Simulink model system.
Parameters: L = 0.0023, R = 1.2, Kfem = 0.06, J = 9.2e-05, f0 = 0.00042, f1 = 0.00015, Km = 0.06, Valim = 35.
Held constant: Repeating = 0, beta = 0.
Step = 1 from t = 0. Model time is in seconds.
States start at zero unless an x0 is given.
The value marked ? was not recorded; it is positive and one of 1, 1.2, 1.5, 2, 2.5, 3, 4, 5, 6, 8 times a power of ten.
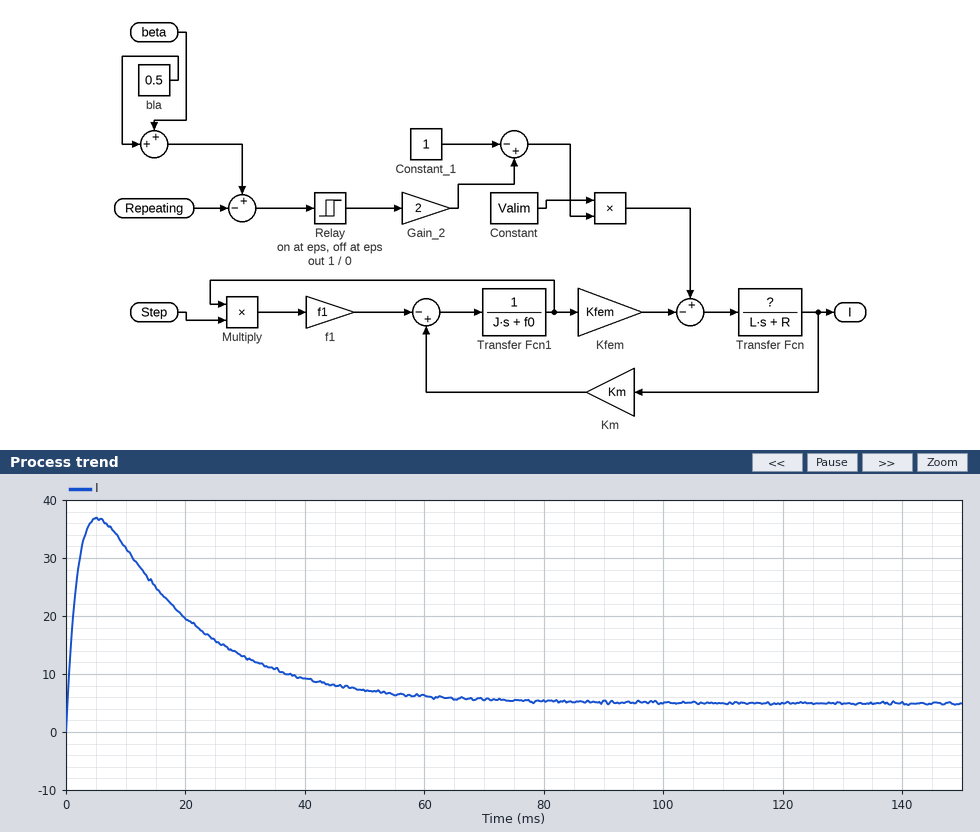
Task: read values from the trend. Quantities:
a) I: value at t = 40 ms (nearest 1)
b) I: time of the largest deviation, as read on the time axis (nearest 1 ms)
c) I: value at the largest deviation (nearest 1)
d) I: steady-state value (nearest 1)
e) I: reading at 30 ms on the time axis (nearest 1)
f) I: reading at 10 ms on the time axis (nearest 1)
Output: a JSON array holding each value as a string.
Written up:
["9", "5 ms", "37", "5", "13", "32"]
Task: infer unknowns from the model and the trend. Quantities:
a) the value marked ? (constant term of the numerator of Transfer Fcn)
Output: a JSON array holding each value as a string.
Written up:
["1.5"]
